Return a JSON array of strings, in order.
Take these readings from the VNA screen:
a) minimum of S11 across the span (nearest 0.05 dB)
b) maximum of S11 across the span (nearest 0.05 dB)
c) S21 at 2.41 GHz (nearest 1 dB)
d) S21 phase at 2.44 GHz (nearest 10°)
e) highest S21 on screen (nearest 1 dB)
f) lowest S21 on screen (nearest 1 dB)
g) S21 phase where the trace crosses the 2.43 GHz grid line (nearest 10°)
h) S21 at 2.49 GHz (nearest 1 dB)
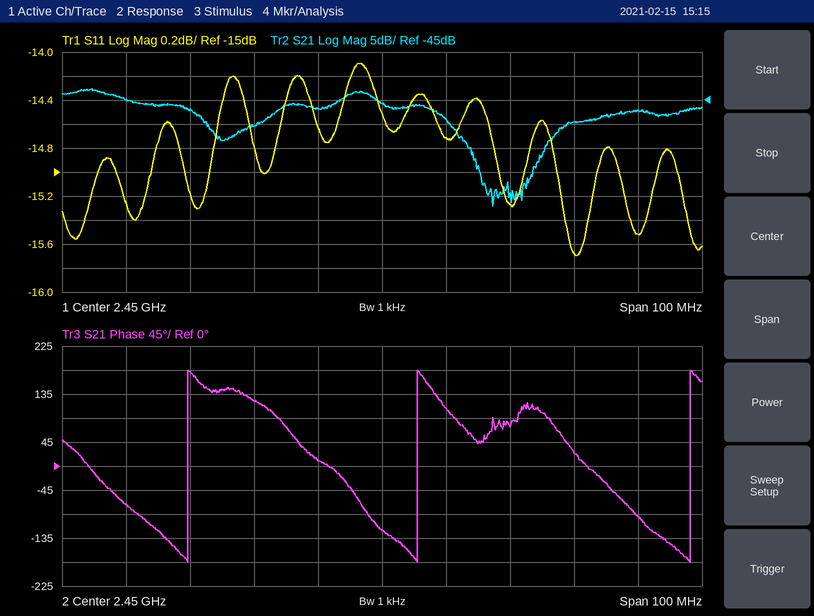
["-15.70 dB", "-14.10 dB", "-45 dB", "10°", "-43 dB", "-67 dB", "120°", "-47 dB"]
